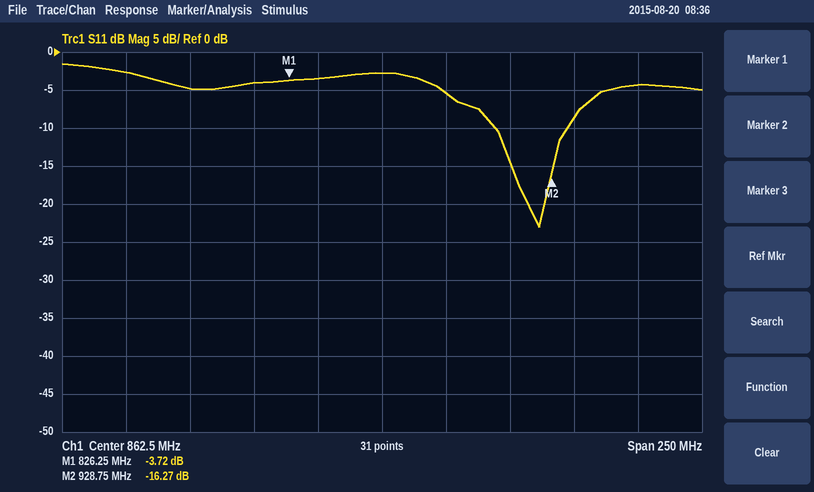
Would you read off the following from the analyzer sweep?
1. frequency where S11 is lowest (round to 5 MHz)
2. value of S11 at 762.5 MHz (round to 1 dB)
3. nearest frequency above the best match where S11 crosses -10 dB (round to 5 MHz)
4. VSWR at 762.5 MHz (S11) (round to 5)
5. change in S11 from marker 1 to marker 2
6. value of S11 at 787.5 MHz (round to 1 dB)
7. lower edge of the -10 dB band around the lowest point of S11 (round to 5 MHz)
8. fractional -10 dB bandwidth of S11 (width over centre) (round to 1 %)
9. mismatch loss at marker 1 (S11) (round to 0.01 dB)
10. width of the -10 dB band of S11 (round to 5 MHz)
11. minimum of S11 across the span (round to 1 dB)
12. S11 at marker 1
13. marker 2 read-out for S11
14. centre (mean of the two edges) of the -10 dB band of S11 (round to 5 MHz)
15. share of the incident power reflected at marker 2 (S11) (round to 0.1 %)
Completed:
925 MHz
-3 dB
935 MHz
5
-12.55 dB
-5 dB
905 MHz
3 %
2.40 dB
30 MHz
-23 dB
-3.72 dB
-16.27 dB
920 MHz
2.4 %
